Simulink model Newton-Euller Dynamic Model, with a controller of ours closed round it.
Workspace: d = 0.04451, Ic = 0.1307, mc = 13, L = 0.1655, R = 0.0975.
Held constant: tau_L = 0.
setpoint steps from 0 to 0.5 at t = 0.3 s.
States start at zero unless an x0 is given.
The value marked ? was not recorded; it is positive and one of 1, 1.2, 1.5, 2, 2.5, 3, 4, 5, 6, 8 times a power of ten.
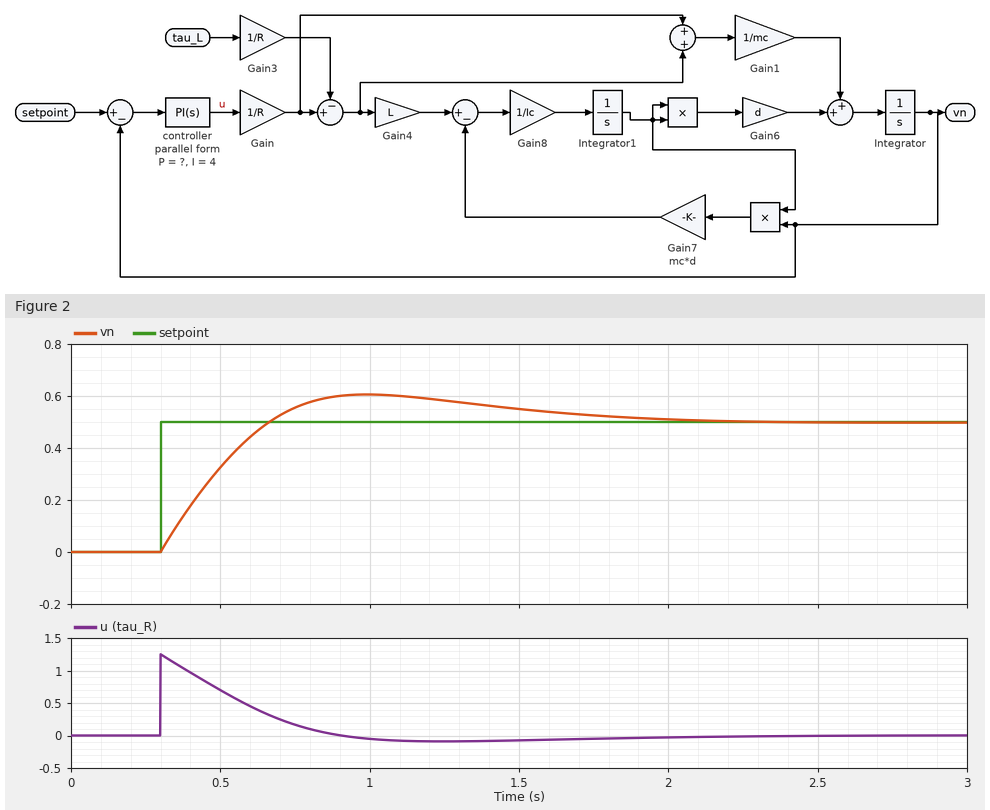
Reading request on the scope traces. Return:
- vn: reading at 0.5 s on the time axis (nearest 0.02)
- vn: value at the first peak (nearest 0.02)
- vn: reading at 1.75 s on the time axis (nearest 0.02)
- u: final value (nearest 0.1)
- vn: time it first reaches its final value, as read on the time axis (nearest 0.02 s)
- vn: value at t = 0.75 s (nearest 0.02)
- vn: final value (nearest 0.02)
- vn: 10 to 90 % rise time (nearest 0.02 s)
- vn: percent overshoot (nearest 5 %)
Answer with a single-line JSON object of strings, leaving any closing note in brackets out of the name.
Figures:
{"vn: reading at 0.5 s on the time axis": "0.32", "vn: value at the first peak": "0.60", "vn: reading at 1.75 s on the time axis": "0.52", "u: final value": "0.0", "vn: time it first reaches its final value, as read on the time axis": "0.66 s", "vn: value at t = 0.75 s": "0.56", "vn: final value": "0.50", "vn: 10 to 90 % rise time": "0.28 s", "vn: percent overshoot": "20 %"}
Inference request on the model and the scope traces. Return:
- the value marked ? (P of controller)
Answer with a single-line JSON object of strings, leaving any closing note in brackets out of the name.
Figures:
{"the value marked ?": "2.5"}
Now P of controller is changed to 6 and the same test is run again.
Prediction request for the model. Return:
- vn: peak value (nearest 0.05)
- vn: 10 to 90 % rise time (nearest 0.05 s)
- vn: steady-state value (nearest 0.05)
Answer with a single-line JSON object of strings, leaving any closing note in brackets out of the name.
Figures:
{"vn: peak value": "0.55", "vn: 10 to 90 % rise time": "0.15 s", "vn: steady-state value": "0.50"}
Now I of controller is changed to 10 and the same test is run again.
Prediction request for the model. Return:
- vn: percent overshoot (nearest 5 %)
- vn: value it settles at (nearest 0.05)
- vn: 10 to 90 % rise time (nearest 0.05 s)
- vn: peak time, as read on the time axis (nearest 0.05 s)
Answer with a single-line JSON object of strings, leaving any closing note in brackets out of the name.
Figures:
{"vn: percent overshoot": "35 %", "vn: value it settles at": "0.50", "vn: 10 to 90 % rise time": "0.20 s", "vn: peak time, as read on the time axis": "0.85 s"}
